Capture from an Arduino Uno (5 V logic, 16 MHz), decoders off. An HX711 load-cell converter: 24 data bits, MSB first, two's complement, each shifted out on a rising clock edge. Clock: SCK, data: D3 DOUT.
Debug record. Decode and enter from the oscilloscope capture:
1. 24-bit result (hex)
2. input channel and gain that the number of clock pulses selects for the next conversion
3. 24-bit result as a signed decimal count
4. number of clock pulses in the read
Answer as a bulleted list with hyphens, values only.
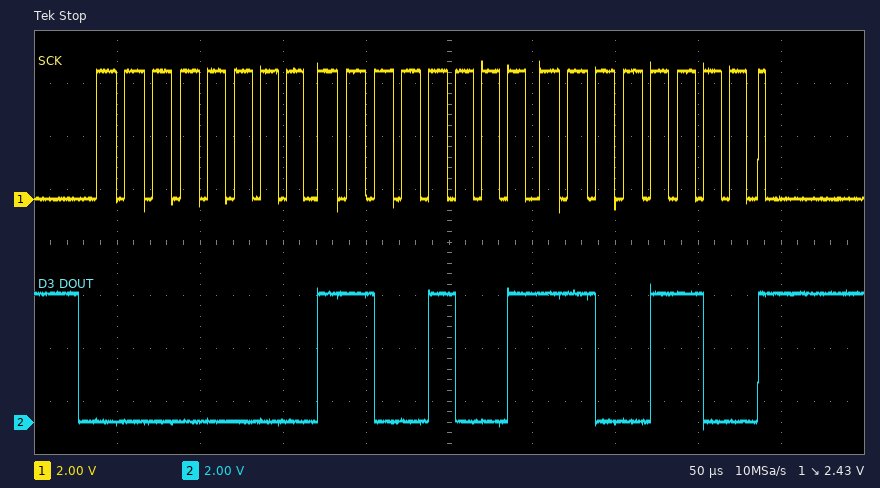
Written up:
- 0x00C9CC
- channel A, gain 128
- 51660
- 25
